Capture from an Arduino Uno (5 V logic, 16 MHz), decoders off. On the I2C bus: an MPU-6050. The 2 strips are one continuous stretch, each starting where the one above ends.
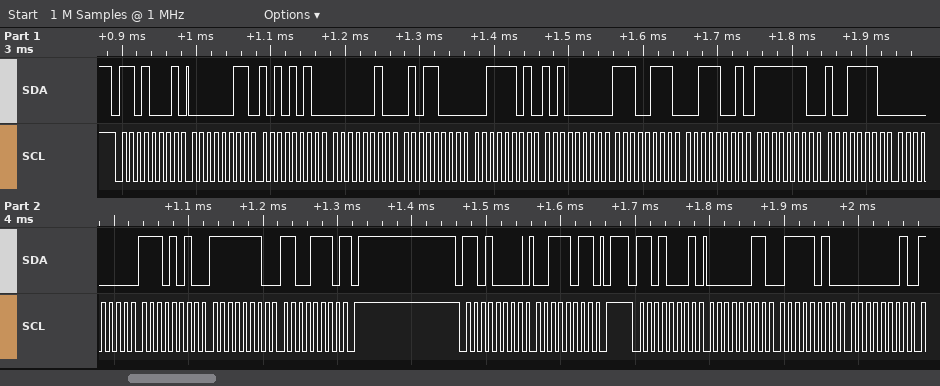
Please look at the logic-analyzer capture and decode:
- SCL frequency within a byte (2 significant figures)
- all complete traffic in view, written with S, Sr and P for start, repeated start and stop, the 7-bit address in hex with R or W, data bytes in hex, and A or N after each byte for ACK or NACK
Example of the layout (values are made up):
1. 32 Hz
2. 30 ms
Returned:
1. 100 kHz
2. S 68R A 03 A AA A 02 A 58 A 3D A A0 A E7 A 39 A FE A 9E A 00 A EA A FE A CE N P S 68W A 3B A P S 68R A 03 A 7A A 01 A
